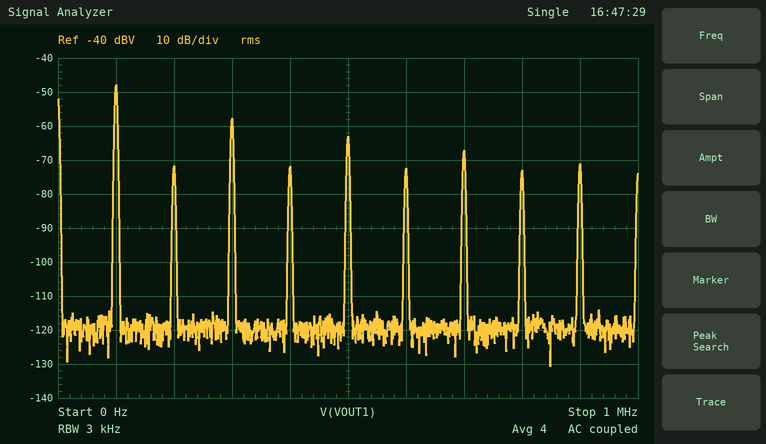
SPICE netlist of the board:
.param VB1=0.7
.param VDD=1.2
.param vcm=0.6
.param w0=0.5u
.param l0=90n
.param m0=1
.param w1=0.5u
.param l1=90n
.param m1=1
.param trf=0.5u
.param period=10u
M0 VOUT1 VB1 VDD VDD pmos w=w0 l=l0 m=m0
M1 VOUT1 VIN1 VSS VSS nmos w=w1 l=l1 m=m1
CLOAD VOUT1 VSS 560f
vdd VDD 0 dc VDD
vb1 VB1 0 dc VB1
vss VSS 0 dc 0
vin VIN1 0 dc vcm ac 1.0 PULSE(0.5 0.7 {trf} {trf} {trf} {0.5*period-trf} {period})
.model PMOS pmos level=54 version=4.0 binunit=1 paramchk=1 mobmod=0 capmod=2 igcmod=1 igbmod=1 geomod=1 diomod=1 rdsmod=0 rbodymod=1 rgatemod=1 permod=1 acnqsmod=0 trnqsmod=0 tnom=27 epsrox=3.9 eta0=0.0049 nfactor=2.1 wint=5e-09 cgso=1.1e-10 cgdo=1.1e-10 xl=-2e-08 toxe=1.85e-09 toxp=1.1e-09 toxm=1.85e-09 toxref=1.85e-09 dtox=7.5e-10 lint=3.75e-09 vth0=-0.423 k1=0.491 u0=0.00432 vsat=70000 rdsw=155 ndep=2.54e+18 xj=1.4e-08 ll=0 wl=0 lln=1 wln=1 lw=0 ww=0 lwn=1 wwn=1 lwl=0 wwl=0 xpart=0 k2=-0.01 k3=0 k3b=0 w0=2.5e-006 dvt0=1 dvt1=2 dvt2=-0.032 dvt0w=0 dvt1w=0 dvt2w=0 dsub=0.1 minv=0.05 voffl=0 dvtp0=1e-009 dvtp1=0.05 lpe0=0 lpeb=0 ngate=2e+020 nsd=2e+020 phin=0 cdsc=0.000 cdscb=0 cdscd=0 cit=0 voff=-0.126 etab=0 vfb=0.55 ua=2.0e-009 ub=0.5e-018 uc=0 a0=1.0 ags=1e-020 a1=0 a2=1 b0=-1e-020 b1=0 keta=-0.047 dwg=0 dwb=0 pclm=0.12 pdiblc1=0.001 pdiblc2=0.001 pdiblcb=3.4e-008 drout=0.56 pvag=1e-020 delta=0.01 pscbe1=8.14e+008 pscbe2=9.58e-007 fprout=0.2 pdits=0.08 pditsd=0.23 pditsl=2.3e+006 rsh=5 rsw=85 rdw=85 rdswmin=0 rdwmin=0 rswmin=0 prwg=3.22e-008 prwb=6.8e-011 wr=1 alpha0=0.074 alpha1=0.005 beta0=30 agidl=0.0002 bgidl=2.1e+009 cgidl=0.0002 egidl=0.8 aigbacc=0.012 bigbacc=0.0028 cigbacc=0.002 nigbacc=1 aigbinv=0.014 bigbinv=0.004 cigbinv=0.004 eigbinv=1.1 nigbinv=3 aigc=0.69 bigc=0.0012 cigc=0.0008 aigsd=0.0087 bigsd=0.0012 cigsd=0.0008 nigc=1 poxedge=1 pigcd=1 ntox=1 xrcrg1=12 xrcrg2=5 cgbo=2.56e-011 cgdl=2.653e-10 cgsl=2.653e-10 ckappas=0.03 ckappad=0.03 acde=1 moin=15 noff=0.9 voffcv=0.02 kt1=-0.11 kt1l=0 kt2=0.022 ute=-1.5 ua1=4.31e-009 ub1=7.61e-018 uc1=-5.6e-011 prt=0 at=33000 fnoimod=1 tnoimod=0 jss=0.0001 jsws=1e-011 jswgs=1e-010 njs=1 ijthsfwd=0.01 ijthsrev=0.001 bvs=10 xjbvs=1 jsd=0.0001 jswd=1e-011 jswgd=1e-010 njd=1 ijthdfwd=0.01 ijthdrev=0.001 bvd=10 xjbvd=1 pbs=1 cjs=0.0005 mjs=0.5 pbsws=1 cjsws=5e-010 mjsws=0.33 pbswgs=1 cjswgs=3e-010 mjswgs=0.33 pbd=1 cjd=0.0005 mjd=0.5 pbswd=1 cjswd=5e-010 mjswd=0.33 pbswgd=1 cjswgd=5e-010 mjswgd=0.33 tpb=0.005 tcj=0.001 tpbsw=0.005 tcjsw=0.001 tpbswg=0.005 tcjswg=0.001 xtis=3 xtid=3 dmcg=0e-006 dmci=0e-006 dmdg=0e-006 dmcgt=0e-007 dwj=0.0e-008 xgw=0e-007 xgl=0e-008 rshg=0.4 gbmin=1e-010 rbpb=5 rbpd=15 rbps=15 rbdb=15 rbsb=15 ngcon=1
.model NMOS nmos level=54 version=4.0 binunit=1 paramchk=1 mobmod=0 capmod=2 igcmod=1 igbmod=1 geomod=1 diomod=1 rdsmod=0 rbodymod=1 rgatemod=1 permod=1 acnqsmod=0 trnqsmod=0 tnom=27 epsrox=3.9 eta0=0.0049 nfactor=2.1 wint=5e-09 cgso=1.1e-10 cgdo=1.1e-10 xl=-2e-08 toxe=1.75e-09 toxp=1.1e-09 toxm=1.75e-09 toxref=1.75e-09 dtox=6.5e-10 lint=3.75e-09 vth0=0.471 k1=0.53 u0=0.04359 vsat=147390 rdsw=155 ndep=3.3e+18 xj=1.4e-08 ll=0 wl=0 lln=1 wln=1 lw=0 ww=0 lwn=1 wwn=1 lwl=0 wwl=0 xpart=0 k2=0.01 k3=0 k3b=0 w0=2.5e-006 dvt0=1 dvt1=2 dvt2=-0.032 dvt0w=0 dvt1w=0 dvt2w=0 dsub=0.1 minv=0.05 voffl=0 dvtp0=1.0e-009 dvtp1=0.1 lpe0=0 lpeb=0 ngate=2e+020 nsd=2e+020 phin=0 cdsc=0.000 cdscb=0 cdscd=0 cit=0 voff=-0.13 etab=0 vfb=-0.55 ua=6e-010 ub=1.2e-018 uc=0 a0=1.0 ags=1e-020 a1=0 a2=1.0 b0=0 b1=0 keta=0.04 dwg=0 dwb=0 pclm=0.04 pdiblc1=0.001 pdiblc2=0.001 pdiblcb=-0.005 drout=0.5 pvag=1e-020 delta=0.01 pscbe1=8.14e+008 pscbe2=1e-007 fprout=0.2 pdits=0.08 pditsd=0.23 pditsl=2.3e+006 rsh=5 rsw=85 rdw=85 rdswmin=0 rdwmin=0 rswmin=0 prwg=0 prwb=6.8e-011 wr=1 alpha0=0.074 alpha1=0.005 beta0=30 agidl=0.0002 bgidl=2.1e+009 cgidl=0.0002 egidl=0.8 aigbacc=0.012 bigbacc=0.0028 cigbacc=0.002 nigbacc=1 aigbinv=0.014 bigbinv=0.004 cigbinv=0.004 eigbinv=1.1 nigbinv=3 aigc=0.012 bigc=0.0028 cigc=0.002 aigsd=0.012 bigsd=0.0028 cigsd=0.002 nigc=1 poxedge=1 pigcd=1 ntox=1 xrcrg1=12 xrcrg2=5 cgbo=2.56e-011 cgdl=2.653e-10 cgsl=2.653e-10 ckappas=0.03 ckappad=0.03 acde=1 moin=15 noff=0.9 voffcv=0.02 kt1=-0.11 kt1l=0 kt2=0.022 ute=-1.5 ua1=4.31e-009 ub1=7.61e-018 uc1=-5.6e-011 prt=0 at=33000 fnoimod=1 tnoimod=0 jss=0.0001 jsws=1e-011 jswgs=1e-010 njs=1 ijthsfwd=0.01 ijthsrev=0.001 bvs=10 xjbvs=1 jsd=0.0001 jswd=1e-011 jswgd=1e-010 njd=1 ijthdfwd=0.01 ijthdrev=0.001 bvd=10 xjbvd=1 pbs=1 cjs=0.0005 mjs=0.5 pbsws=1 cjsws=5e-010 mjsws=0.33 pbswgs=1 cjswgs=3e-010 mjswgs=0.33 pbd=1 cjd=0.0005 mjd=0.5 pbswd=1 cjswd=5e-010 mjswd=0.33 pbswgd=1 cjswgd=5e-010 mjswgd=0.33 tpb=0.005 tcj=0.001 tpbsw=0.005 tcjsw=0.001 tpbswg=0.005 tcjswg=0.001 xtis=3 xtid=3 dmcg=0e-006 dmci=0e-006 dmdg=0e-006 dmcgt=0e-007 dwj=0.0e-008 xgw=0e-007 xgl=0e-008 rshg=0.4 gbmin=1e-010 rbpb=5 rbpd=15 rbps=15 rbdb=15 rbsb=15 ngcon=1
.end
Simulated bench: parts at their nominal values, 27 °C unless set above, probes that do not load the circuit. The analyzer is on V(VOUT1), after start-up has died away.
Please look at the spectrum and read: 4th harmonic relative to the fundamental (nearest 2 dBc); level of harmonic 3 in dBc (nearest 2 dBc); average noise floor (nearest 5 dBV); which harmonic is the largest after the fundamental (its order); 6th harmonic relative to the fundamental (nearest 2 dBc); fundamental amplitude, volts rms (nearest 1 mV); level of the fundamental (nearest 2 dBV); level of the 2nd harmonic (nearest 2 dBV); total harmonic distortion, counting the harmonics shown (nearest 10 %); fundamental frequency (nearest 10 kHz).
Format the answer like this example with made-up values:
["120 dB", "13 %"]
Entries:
["-24 dBc", "-10 dBc", "-120 dBV", "3", "-24 dBc", "4 mV", "-48 dBV", "-72 dBV", "40 %", "100 kHz"]
